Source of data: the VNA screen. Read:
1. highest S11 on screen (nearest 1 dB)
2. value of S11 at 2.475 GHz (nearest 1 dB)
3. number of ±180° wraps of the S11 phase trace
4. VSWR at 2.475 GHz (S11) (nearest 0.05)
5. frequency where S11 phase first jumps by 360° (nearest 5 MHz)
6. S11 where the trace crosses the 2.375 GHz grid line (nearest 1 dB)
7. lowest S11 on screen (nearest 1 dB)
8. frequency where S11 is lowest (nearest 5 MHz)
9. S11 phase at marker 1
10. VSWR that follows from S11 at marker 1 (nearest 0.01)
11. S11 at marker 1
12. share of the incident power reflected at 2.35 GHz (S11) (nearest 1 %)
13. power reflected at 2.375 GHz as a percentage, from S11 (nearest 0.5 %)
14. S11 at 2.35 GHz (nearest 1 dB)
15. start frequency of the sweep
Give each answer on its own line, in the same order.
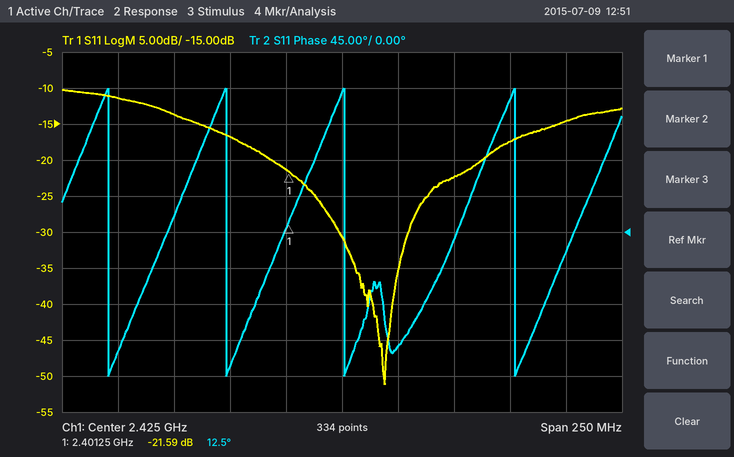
-10 dB
-22 dB
4
1.15
2.320 GHz
-17 dB
-51 dB
2.445 GHz
12.5°
1.18
-21.59 dB
4 %
2.0 %
-14 dB
2.3 GHz
